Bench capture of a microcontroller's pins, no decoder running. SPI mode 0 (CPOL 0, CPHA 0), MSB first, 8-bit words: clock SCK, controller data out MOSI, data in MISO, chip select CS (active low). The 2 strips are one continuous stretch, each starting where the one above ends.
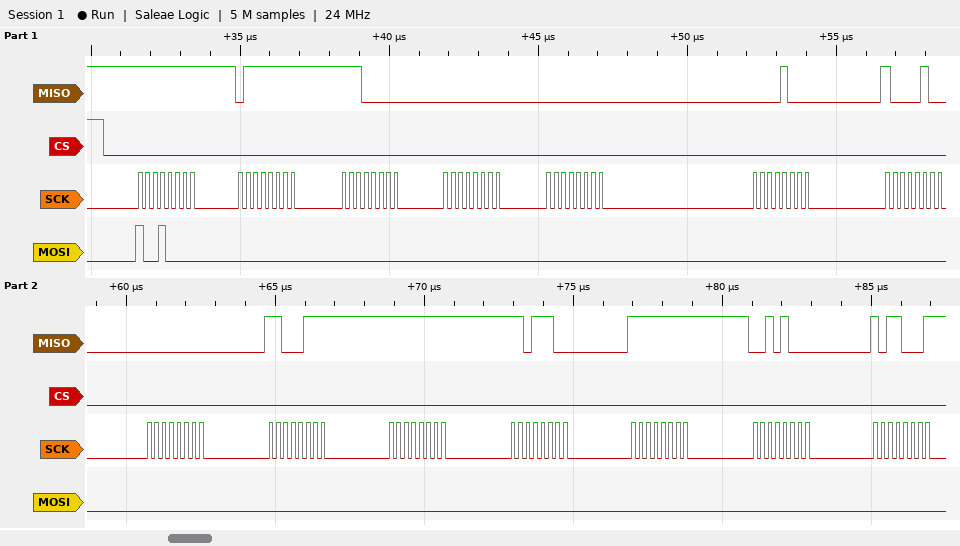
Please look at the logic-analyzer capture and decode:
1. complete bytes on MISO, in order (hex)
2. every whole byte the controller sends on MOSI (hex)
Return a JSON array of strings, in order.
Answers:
["FF 7F E0 00 00 08 84 00 C7 FF DC FF 28 B1", "90 00 00 00 00 00 00 00 00 00 00 00 00 00"]
